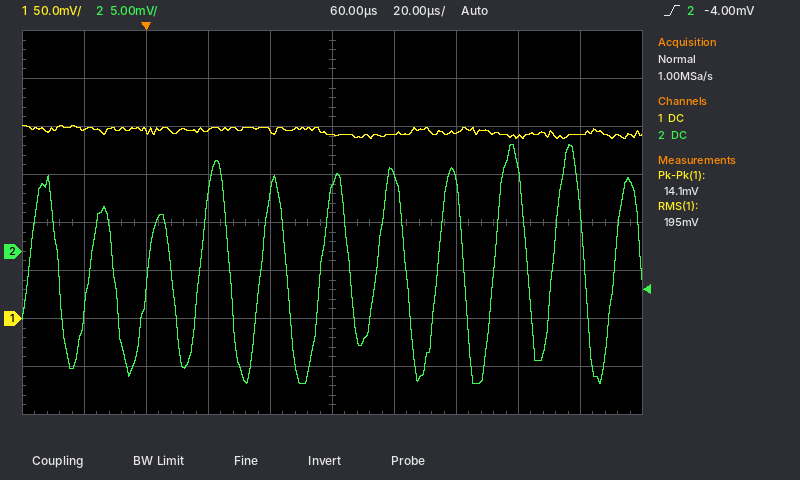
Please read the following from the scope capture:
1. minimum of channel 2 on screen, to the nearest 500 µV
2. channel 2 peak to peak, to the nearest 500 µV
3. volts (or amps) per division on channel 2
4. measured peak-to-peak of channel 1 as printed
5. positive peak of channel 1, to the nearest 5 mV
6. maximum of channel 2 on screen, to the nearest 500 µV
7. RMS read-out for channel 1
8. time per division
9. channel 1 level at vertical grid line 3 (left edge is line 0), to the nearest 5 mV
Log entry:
-14.0 mV
25.0 mV
5 mV
14.1 mV
200 mV
11.0 mV
195 mV
20 µs
195 mV
